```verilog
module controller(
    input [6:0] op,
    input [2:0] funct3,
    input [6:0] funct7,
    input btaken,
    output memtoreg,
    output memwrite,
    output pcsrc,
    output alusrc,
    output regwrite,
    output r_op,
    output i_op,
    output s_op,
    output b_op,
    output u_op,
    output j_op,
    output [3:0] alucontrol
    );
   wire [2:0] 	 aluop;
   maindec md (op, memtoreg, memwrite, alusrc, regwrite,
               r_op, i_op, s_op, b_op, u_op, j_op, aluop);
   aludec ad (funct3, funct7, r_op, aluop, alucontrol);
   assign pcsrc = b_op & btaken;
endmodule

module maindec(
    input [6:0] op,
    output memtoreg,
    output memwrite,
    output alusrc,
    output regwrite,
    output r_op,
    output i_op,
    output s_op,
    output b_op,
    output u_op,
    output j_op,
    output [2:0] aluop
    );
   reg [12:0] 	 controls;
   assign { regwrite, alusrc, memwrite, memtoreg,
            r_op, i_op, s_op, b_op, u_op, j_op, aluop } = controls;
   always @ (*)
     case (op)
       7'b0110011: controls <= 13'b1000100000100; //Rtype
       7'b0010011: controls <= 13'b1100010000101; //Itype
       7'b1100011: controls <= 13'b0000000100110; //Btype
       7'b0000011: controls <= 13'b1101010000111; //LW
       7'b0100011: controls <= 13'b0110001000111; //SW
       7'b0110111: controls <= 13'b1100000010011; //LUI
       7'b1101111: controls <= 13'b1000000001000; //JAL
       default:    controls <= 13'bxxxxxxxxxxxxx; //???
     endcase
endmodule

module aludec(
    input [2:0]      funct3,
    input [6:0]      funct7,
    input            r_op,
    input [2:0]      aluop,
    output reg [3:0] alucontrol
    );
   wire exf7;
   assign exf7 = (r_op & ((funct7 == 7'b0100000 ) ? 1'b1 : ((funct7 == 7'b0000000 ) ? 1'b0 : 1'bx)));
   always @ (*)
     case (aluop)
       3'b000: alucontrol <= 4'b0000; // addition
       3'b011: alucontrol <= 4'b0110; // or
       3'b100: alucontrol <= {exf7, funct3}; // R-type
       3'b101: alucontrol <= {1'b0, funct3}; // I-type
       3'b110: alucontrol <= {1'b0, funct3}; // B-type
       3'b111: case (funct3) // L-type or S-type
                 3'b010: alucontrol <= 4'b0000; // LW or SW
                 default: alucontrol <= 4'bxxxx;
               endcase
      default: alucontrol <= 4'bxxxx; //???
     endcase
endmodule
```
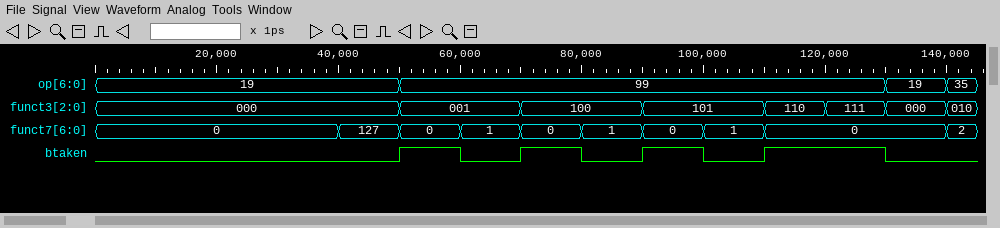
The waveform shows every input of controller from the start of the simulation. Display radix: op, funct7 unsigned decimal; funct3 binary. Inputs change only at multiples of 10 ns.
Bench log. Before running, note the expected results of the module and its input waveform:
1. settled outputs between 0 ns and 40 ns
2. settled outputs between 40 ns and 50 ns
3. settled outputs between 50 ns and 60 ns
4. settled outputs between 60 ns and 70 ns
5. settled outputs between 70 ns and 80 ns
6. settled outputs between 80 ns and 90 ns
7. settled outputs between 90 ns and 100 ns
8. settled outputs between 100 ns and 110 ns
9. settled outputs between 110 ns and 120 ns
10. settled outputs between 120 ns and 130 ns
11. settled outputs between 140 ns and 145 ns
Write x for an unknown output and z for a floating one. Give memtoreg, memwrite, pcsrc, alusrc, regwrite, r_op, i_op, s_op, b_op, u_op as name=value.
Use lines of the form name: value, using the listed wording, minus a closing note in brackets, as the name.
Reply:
settled outputs between 0 ns and 40 ns: memtoreg=0, memwrite=0, pcsrc=0, alusrc=1, regwrite=1, r_op=0, i_op=1, s_op=0, b_op=0, u_op=0
settled outputs between 40 ns and 50 ns: memtoreg=0, memwrite=0, pcsrc=0, alusrc=1, regwrite=1, r_op=0, i_op=1, s_op=0, b_op=0, u_op=0
settled outputs between 50 ns and 60 ns: memtoreg=0, memwrite=0, pcsrc=1, alusrc=0, regwrite=0, r_op=0, i_op=0, s_op=0, b_op=1, u_op=0
settled outputs between 60 ns and 70 ns: memtoreg=0, memwrite=0, pcsrc=0, alusrc=0, regwrite=0, r_op=0, i_op=0, s_op=0, b_op=1, u_op=0
settled outputs between 70 ns and 80 ns: memtoreg=0, memwrite=0, pcsrc=1, alusrc=0, regwrite=0, r_op=0, i_op=0, s_op=0, b_op=1, u_op=0
settled outputs between 80 ns and 90 ns: memtoreg=0, memwrite=0, pcsrc=0, alusrc=0, regwrite=0, r_op=0, i_op=0, s_op=0, b_op=1, u_op=0
settled outputs between 90 ns and 100 ns: memtoreg=0, memwrite=0, pcsrc=1, alusrc=0, regwrite=0, r_op=0, i_op=0, s_op=0, b_op=1, u_op=0
settled outputs between 100 ns and 110 ns: memtoreg=0, memwrite=0, pcsrc=0, alusrc=0, regwrite=0, r_op=0, i_op=0, s_op=0, b_op=1, u_op=0
settled outputs between 110 ns and 120 ns: memtoreg=0, memwrite=0, pcsrc=1, alusrc=0, regwrite=0, r_op=0, i_op=0, s_op=0, b_op=1, u_op=0
settled outputs between 120 ns and 130 ns: memtoreg=0, memwrite=0, pcsrc=1, alusrc=0, regwrite=0, r_op=0, i_op=0, s_op=0, b_op=1, u_op=0
settled outputs between 140 ns and 145 ns: memtoreg=0, memwrite=1, pcsrc=0, alusrc=1, regwrite=0, r_op=0, i_op=0, s_op=1, b_op=0, u_op=0
